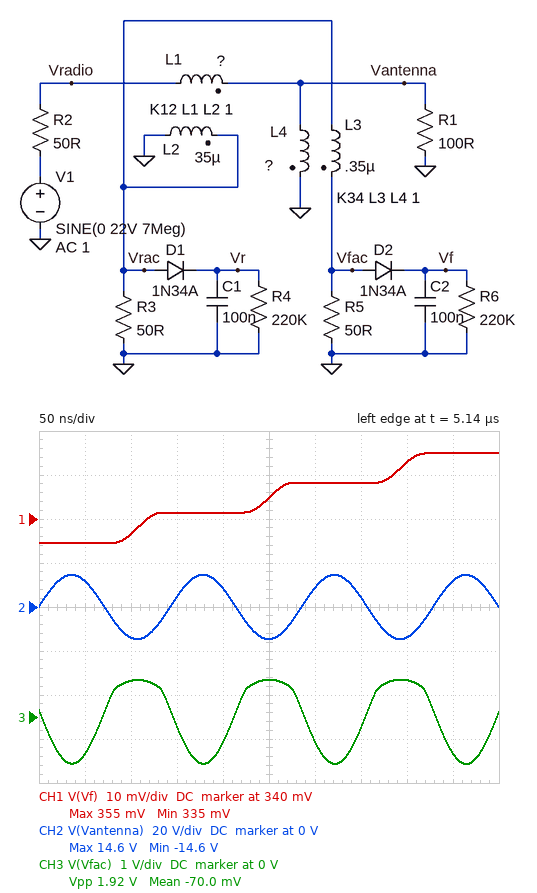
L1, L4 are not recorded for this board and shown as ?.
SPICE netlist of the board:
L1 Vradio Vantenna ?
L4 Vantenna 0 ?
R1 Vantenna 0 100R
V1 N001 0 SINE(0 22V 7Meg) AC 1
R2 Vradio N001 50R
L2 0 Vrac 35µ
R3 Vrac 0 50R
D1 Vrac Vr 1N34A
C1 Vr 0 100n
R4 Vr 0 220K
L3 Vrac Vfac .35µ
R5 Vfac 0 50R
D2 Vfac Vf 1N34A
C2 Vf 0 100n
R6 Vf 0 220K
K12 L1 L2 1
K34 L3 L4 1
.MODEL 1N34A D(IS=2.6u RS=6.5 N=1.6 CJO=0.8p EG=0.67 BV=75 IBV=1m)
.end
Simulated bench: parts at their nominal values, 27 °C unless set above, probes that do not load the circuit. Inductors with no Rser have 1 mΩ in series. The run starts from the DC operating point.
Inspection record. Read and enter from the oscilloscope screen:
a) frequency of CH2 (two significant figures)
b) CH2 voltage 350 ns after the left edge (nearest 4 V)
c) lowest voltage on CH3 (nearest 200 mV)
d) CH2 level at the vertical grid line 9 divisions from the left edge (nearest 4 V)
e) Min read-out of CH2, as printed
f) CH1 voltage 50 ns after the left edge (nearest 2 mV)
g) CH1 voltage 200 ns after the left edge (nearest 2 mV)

7.0 MHz
4 V
-1.0 V
12 V
-14.6 V
334 mV
342 mV
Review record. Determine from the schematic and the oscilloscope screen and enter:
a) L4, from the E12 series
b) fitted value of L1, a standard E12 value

56 µH
1 µH
